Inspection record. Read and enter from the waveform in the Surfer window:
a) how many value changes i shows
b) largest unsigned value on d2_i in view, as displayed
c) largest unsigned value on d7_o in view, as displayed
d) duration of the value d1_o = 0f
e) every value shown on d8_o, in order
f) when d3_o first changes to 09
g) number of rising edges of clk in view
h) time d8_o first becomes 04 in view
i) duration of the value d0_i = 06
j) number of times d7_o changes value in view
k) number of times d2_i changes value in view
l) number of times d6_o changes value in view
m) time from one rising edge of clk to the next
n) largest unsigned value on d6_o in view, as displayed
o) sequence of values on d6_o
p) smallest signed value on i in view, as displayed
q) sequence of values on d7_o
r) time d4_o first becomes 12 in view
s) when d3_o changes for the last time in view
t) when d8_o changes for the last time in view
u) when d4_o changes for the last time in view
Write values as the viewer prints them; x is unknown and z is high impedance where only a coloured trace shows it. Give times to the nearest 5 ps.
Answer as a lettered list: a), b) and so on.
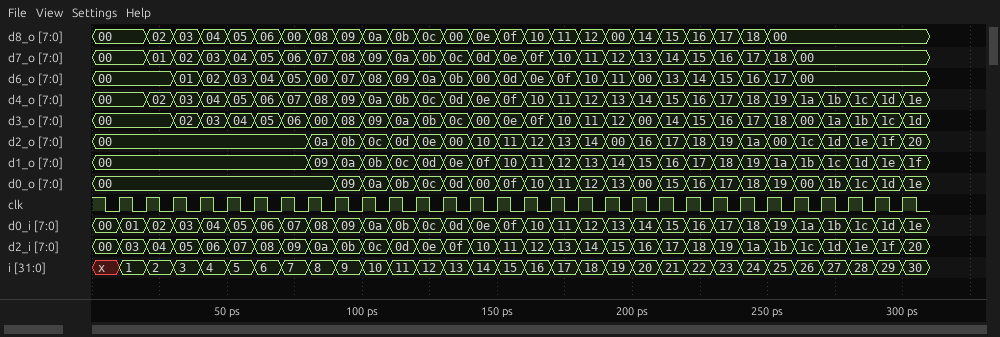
a) 30
b) 20
c) 18
d) 10 ps
e) 00, 02, 03, 04, 05, 06, 00, 08, 09, 0a, 0b, 0c, 00, 0e, 0f, 10, 11, 12, 00, 14, 15, 16, 17, 18, 00
f) 100 ps
g) 30
h) 40 ps
i) 10 ps
j) 25
k) 30
l) 24
m) 10 ps
n) 17
o) 00, 01, 02, 03, 04, 05, 00, 07, 08, 09, 0a, 0b, 00, 0d, 0e, 0f, 10, 11, 00, 13, 14, 15, 16, 17, 00
p) 1
q) 00, 01, 02, 03, 04, 05, 06, 07, 08, 09, 0a, 0b, 0c, 0d, 0e, 0f, 10, 11, 12, 13, 14, 15, 16, 17, 18, 00
r) 180 ps
s) 300 ps
t) 250 ps
u) 300 ps
